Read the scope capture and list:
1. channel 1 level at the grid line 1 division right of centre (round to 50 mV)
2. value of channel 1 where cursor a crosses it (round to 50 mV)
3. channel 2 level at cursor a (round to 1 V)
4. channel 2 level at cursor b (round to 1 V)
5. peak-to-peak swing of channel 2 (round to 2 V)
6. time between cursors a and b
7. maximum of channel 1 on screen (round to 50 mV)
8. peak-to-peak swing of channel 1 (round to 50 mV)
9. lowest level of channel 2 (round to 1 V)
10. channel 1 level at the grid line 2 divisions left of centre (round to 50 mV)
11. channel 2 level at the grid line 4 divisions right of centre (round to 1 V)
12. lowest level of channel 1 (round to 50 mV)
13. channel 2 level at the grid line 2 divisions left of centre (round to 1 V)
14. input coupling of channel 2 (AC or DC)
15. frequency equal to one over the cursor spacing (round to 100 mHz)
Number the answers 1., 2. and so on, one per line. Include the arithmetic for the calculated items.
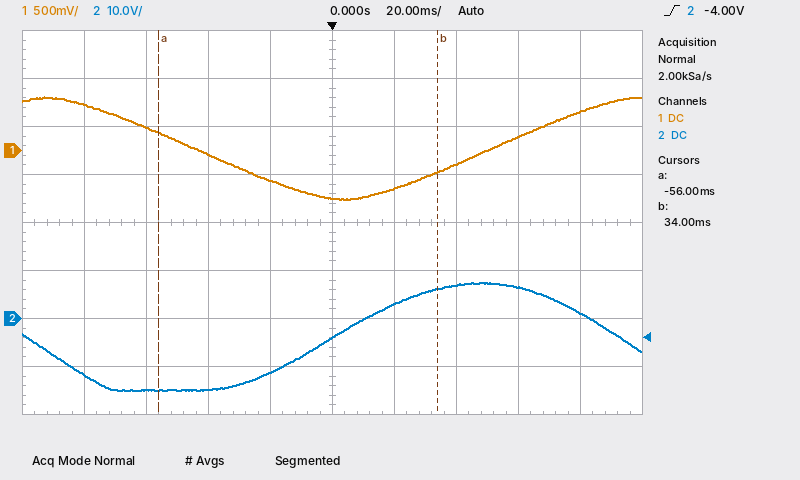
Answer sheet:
1. -400 mV
2. 200 mV
3. -15 V
4. 6 V
5. 22 V
6. 34 ms − (-56 ms) = 90 ms
7. 550 mV
8. 550 mV − (-500 mV) = 1.05 V
9. -15 V
10. -50 mV
11. 1 V
12. -500 mV
13. -15 V
14. DC
15. 1 / 90 ms ≈ 11.1 Hz
